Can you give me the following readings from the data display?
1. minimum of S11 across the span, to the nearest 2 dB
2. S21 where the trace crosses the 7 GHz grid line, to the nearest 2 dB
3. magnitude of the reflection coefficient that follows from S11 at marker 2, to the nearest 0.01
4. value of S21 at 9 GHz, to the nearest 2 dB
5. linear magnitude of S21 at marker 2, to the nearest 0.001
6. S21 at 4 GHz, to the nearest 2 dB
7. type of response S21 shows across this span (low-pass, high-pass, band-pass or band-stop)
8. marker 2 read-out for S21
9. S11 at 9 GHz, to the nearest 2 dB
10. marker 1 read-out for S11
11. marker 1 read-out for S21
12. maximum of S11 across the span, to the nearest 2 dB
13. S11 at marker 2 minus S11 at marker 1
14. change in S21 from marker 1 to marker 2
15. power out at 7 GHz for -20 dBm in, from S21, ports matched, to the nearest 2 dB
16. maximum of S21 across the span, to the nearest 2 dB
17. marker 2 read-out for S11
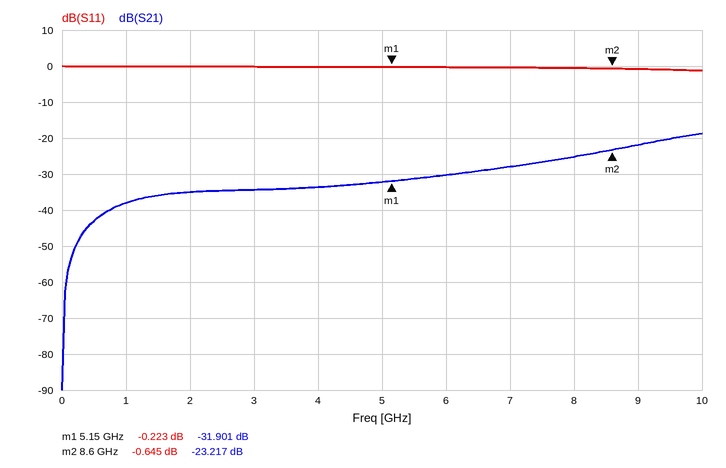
-2 dB
-28 dB
0.93
-22 dB
0.069
-34 dB
high-pass
-23.217 dB
0 dB
-0.223 dB
-31.901 dB
0 dB
-0.422 dB
8.684 dB
-48 dBm
-18 dB
-0.645 dB
